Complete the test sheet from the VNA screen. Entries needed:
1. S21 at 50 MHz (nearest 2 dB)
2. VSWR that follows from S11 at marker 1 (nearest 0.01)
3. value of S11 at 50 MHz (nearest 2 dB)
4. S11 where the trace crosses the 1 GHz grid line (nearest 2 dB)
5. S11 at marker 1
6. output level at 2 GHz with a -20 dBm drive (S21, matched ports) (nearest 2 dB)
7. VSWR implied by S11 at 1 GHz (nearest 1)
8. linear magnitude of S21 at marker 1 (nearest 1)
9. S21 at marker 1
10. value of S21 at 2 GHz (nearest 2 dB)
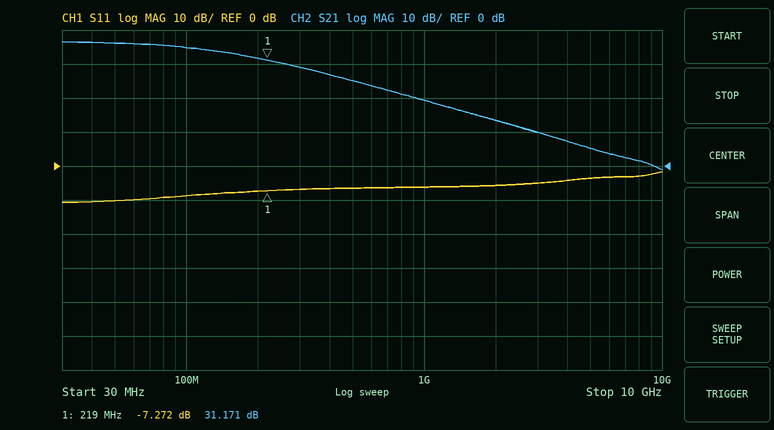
36 dB
2.53
-10 dB
-6 dB
-7.272 dB
-6 dBm
3
36
31.171 dB
14 dB
